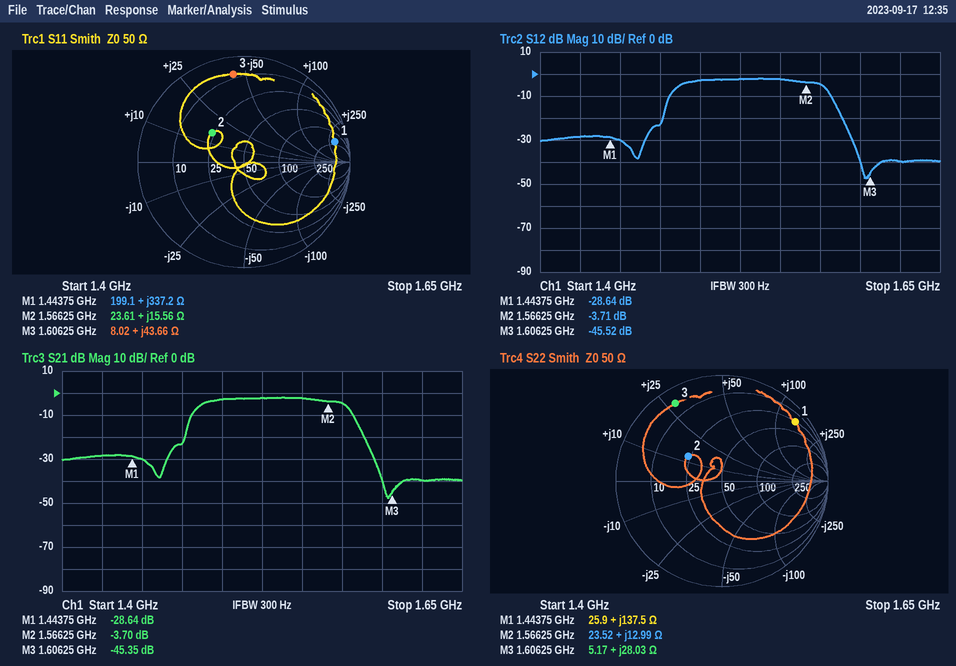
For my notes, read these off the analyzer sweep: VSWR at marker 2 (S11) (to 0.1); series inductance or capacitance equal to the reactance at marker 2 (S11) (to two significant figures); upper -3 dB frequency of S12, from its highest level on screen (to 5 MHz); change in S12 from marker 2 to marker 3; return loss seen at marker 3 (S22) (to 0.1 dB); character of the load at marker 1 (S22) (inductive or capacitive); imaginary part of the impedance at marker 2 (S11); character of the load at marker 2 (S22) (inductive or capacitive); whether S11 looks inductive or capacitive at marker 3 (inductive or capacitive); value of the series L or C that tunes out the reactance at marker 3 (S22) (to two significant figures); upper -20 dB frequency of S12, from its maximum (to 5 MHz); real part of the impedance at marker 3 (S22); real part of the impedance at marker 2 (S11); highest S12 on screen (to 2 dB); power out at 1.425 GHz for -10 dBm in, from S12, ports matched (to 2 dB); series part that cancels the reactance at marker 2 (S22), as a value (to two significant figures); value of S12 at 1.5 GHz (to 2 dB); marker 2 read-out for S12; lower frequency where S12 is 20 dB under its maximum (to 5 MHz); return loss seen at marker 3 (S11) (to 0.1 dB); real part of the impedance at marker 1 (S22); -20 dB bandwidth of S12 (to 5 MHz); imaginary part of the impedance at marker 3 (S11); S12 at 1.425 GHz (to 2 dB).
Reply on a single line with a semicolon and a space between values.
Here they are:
2.4; 1.6 nH; 1.575 GHz; -41.81 dB; 1.4 dB; inductive; +15.56 Ω; inductive; inductive; 3.5 pF; 1.590 GHz; 5.17 Ω; 23.61 Ω; -2 dB; -38 dBm; 7.8 pF; -2 dB; -3.71 dB; 1.475 GHz; 1.6 dB; 25.9 Ω; 115 MHz; +43.66 Ω; -28 dB
